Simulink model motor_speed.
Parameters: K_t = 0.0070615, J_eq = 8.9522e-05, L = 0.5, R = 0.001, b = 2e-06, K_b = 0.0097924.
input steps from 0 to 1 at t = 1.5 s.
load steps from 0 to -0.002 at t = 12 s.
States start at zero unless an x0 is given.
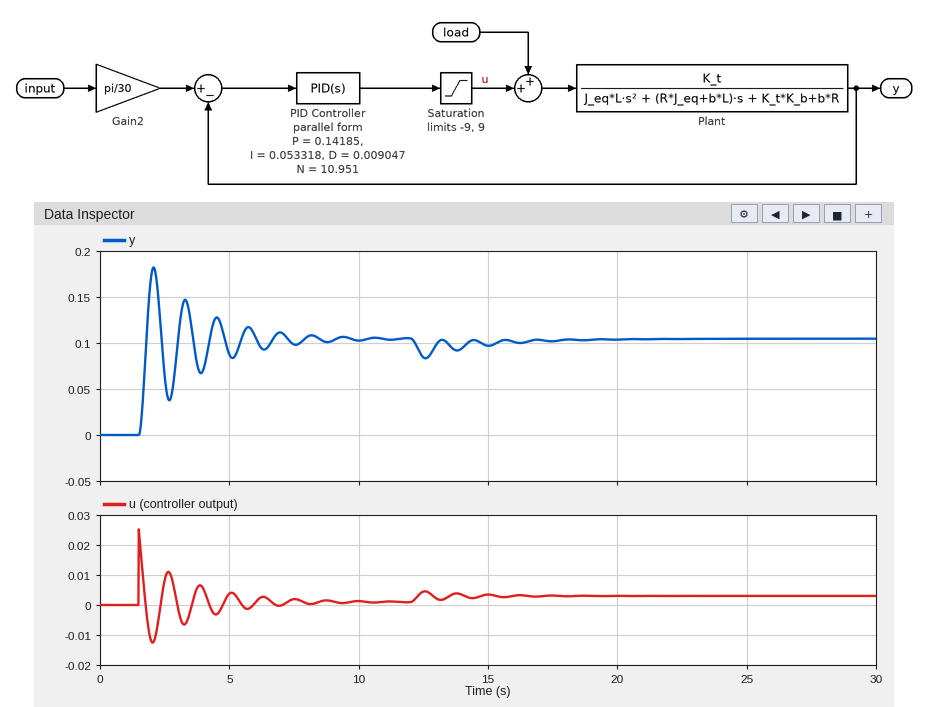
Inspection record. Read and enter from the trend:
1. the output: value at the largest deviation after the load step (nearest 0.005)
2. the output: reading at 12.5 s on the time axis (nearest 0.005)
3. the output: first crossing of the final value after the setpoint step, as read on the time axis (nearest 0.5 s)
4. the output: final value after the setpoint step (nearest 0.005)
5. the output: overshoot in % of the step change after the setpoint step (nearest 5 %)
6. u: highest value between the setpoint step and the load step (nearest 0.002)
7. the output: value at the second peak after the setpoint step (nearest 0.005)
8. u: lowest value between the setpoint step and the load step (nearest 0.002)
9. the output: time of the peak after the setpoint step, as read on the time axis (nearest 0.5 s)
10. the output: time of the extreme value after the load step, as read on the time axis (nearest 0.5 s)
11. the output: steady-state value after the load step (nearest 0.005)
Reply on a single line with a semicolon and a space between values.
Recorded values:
0.085; 0.085; 2.0 s; 0.105; 75 %; 0.026; 0.145; -0.012; 2.0 s; 12.5 s; 0.105
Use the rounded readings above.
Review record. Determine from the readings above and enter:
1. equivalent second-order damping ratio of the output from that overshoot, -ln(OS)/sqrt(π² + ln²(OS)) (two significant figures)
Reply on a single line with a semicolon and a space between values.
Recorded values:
0.091
